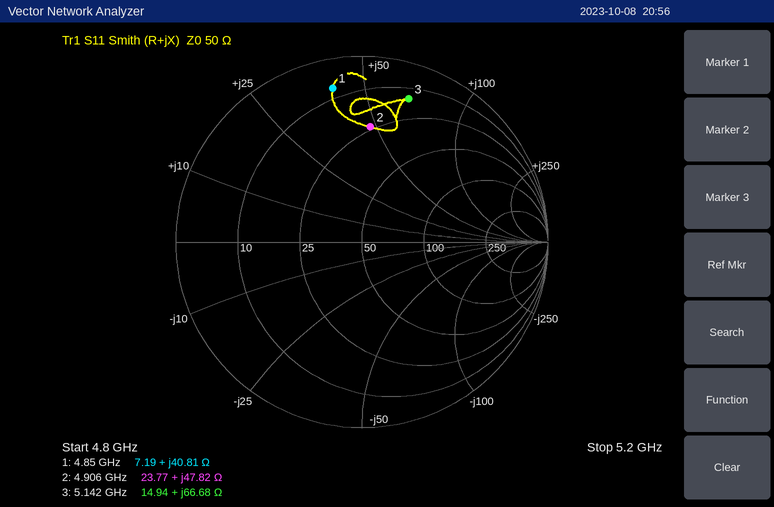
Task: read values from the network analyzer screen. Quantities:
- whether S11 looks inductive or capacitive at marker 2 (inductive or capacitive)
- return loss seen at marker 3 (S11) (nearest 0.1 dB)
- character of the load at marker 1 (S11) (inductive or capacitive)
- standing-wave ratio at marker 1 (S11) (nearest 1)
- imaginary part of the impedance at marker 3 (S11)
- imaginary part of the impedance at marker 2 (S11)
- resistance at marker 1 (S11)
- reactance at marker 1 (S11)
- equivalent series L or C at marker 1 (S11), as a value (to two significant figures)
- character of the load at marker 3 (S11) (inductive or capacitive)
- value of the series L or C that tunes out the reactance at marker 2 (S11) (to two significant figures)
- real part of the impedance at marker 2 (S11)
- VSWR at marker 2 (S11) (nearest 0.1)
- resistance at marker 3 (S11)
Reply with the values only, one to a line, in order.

inductive
1.8 dB
inductive
12
+66.68 Ω
+47.82 Ω
7.19 Ω
+40.81 Ω
1.3 nH
inductive
680 fF
23.77 Ω
4.3
14.94 Ω
